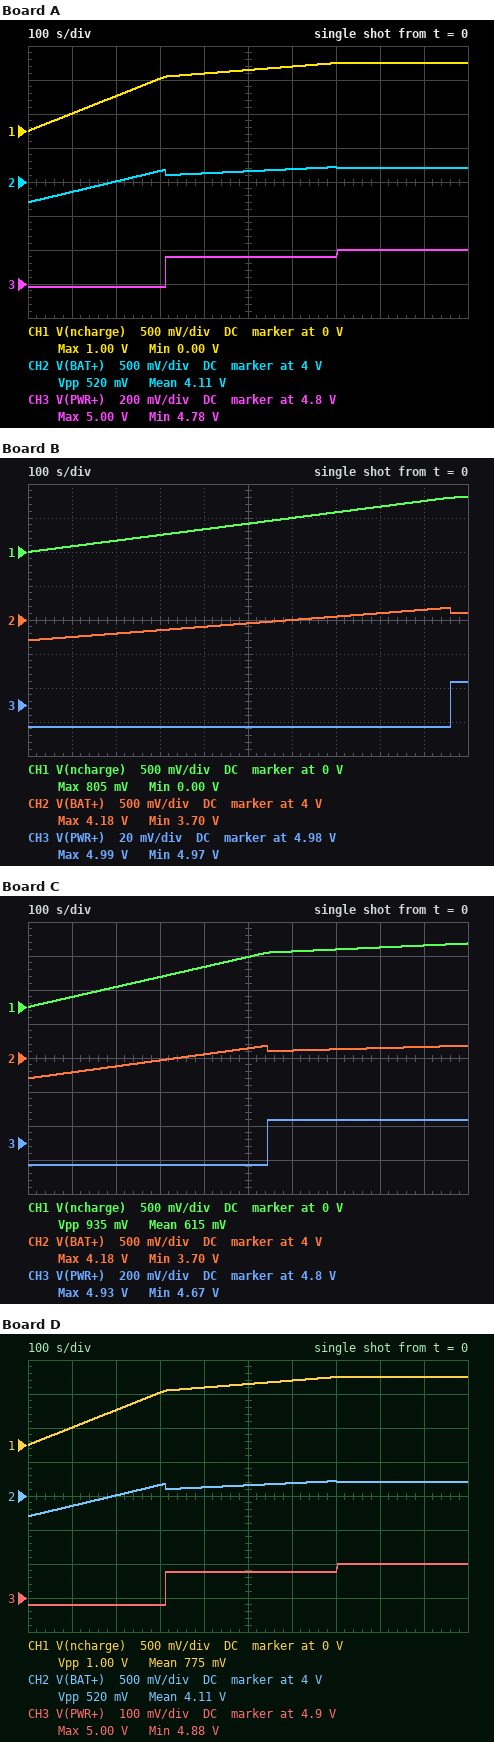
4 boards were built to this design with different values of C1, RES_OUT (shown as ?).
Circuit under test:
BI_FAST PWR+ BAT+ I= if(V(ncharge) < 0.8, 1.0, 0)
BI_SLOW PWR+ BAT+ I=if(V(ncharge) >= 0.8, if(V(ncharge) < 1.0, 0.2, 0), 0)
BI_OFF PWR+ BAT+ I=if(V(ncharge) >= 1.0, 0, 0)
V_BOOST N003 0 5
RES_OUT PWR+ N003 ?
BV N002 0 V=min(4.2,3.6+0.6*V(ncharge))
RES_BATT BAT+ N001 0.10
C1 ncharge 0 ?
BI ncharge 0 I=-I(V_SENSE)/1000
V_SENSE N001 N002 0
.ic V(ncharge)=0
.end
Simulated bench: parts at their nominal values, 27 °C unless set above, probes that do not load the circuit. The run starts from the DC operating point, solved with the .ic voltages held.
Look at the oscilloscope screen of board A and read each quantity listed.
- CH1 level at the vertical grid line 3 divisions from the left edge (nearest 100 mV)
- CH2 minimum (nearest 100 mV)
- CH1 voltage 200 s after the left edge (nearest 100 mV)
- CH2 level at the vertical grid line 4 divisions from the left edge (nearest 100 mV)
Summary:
800 mV
3.7 V
500 mV
4.1 V
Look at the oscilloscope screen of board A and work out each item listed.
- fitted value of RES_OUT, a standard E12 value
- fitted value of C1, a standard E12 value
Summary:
0.22 Ω
390 mF
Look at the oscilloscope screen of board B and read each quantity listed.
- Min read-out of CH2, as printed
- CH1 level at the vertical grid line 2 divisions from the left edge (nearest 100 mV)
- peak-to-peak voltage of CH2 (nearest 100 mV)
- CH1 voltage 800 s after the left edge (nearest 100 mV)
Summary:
3.70 V
200 mV
500 mV
700 mV
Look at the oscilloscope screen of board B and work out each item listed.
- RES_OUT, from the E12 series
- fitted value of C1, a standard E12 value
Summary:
0.033 Ω
1.2 F
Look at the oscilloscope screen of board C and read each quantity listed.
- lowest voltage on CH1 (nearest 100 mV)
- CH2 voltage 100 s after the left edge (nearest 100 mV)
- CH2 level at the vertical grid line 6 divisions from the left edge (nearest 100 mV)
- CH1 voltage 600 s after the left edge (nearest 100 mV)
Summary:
0 V
3.8 V
4.1 V
800 mV
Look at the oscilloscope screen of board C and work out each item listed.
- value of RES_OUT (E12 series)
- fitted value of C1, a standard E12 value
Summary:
0.33 Ω
680 mF
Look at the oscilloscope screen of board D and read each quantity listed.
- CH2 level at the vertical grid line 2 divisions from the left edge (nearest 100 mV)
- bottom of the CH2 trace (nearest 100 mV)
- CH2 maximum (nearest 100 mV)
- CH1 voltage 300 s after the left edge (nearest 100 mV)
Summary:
4.0 V
3.7 V
4.2 V
800 mV
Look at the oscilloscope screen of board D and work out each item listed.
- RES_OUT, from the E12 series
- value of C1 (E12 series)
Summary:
0.12 Ω
390 mF
